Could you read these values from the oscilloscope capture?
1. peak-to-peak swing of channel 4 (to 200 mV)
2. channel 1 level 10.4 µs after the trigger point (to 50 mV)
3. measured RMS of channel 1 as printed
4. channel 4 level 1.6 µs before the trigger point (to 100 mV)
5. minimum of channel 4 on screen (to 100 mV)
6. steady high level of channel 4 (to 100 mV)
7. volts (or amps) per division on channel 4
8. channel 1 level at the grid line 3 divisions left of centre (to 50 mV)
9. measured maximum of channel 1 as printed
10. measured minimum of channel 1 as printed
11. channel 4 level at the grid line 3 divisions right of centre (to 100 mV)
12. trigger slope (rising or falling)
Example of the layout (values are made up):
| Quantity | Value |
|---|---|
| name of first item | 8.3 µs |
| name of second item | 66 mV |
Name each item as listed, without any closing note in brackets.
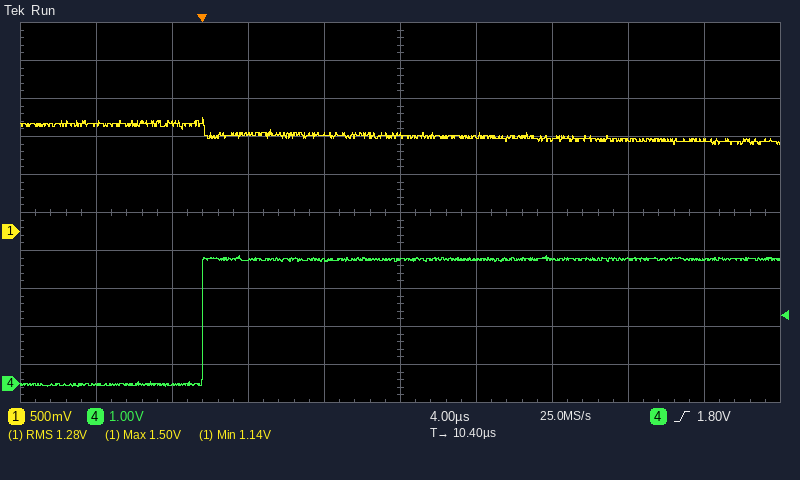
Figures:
| Quantity | Value |
|---|---|
| peak-to-peak swing of channel 4 | 3.4 V |
| channel 1 level 10.4 µs after the trigger point | 1.25 V |
| measured RMS of channel 1 as printed | 1.28 V |
| channel 4 level 1.6 µs before the trigger point | 0.0 V |
| minimum of channel 4 on screen | -100 mV |
| steady high level of channel 4 | 3.3 V |
| volts (or amps) per division on channel 4 | 1 V |
| channel 1 level at the grid line 3 divisions left of centre | 1.40 V |
| measured maximum of channel 1 as printed | 1.50 V |
| measured minimum of channel 1 as printed | 1.14 V |
| channel 4 level at the grid line 3 divisions right of centre | 3.3 V |
| trigger slope | rising |
